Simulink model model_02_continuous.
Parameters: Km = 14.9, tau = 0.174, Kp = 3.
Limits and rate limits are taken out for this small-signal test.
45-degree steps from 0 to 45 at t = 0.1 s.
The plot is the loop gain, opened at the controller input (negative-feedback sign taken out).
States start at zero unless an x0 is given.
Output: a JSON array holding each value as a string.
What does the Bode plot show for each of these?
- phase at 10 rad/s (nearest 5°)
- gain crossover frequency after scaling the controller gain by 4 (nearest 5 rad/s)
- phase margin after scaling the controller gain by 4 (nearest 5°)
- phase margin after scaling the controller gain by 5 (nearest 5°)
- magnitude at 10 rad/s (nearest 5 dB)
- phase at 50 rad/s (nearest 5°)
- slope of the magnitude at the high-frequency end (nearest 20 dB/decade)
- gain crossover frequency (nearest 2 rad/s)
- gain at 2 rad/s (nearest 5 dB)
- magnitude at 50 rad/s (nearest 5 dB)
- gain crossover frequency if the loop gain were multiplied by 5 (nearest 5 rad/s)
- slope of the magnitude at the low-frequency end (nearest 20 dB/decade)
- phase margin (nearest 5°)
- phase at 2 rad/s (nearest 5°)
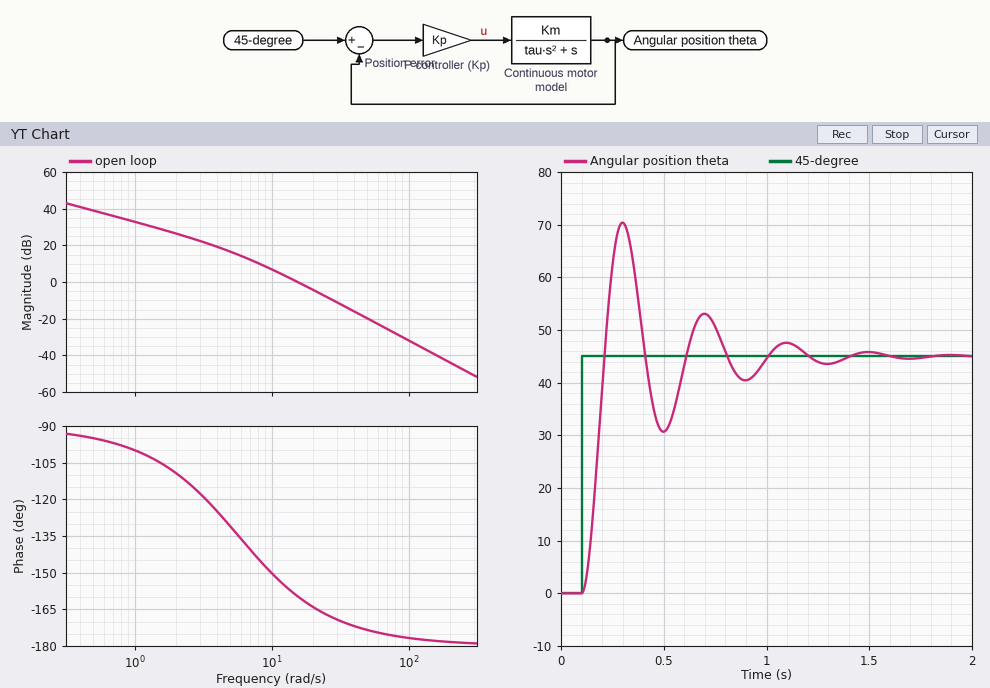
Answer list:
["-150°", "30 rad/s", "10°", "10°", "5 dB", "-175°", "-40 dB/decade", "16 rad/s", "25 dB", "-20 dB", "35 rad/s", "-20 dB/decade", "20°", "-110°"]
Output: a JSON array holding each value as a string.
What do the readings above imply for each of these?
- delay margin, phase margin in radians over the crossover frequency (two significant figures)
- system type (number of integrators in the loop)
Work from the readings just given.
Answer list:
["0.022 s", "1"]
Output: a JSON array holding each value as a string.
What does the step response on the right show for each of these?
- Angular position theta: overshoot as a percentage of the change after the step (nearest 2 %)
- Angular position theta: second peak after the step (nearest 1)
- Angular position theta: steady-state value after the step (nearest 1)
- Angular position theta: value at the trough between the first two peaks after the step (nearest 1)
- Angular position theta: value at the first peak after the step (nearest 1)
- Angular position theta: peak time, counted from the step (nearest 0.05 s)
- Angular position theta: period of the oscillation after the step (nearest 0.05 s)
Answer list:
["56 %", "53", "45", "31", "70", "0.20 s", "0.40 s"]
